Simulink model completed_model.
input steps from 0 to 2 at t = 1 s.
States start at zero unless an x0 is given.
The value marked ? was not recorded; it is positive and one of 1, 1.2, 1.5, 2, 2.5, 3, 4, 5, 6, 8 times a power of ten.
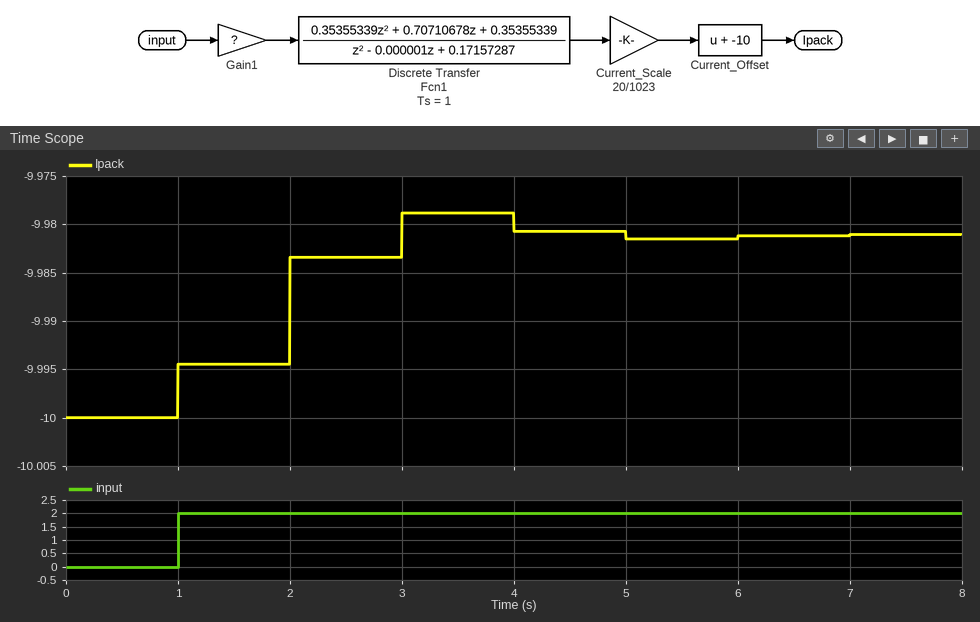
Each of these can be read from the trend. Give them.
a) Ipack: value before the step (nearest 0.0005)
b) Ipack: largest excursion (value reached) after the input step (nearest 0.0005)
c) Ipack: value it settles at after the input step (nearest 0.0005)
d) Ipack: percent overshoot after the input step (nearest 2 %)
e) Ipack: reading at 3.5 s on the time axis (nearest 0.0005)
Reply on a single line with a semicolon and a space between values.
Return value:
-10.0000; -9.9790; -9.9810; 12 %; -9.9790
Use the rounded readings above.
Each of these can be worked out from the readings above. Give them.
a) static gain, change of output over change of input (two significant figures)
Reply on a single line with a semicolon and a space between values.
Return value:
0.0095
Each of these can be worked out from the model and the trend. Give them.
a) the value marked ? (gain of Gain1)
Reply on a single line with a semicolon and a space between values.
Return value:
0.4
